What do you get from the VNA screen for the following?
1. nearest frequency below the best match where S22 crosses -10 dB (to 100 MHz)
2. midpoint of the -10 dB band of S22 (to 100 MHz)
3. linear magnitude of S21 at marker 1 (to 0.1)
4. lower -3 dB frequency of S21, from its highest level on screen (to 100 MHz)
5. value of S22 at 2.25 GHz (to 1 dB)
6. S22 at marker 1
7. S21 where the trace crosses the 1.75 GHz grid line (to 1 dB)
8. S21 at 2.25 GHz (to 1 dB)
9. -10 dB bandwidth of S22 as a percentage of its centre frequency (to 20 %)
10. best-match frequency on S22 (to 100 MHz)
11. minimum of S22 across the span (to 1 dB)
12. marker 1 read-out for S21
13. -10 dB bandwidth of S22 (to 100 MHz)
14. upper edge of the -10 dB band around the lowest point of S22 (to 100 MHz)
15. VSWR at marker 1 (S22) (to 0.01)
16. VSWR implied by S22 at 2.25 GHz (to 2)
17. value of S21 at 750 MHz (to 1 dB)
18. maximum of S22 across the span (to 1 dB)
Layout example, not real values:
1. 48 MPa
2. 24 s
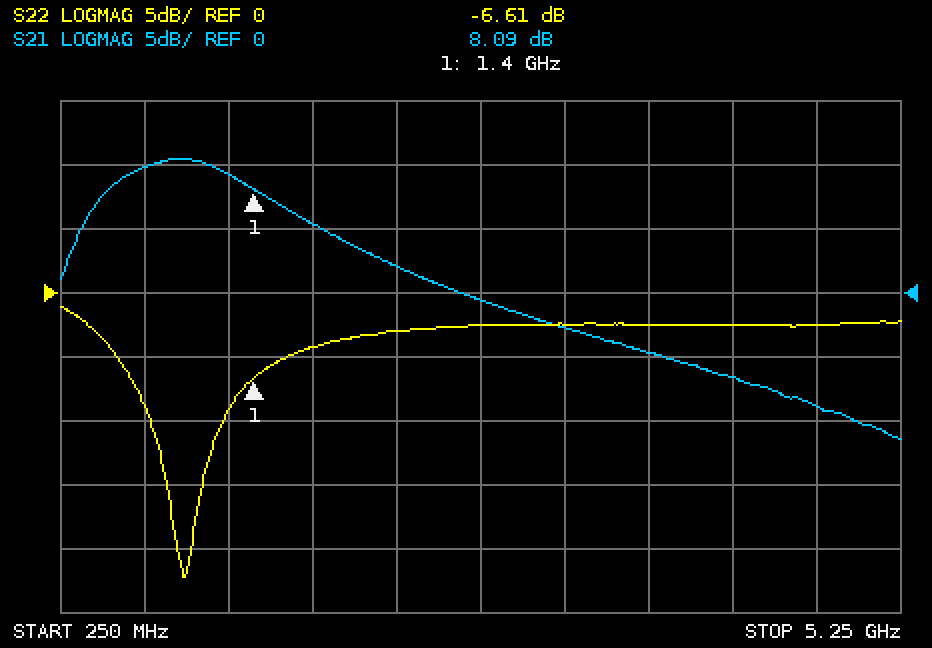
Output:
1. 800 MHz
2. 1.0 GHz
3. 2.5
4. 500 MHz
5. -3 dB
6. -6.61 dB
7. 5 dB
8. 2 dB
9. 40 %
10. 1.0 GHz
11. -22 dB
12. 8.09 dB
13. 400 MHz
14. 1.2 GHz
15. 2.75
16. 6
17. 10 dB
18. -1 dB
